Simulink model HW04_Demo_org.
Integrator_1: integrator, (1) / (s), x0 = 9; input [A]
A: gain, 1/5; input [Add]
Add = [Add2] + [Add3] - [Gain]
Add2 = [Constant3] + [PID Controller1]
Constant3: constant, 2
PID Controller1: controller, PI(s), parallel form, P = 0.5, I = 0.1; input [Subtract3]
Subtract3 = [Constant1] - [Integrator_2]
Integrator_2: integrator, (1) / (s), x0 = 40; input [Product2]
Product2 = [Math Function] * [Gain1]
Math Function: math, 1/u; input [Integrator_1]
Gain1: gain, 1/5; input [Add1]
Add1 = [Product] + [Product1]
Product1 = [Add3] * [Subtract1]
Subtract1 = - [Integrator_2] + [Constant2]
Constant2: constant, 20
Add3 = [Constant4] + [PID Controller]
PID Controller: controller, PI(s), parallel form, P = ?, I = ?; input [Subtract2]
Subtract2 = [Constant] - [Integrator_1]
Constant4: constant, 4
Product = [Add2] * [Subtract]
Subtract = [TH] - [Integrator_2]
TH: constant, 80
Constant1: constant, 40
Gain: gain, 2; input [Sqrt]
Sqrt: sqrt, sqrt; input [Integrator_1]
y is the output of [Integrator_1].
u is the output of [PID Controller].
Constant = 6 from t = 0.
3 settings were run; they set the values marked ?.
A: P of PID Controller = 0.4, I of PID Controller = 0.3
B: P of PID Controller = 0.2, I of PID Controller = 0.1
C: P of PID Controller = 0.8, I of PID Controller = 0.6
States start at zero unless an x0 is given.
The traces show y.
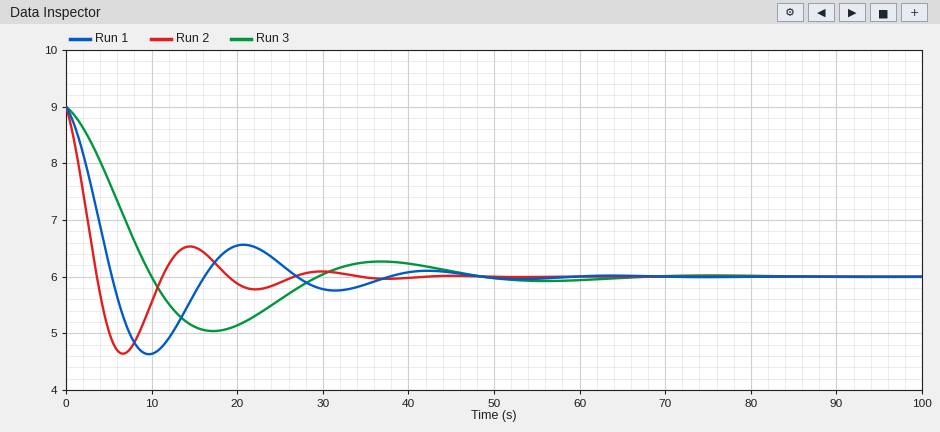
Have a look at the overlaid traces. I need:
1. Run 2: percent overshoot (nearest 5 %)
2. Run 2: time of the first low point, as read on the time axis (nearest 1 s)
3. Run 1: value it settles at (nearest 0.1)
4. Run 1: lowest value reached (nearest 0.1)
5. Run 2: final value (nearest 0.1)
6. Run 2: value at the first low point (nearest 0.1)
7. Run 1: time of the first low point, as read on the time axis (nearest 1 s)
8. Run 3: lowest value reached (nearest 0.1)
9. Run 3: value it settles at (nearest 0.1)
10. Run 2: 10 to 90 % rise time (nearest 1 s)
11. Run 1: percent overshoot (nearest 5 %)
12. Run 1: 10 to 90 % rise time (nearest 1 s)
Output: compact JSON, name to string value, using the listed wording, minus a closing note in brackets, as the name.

{"Run 2: percent overshoot": "45 %", "Run 2: time of the first low point, as read on the time axis": "7 s", "Run 1: value it settles at": "6.0", "Run 1: lowest value reached": "4.6", "Run 2: final value": "6.0", "Run 2: value at the first low point": "4.6", "Run 1: time of the first low point, as read on the time axis": "10 s", "Run 3: lowest value reached": "5.0", "Run 3: value it settles at": "6.0", "Run 2: 10 to 90 % rise time": "3 s", "Run 1: percent overshoot": "45 %", "Run 1: 10 to 90 % rise time": "4 s"}
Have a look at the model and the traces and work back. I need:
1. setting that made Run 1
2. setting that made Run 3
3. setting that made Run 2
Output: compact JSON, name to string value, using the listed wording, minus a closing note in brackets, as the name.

{"setting that made Run 1": "A", "setting that made Run 3": "B", "setting that made Run 2": "C"}
